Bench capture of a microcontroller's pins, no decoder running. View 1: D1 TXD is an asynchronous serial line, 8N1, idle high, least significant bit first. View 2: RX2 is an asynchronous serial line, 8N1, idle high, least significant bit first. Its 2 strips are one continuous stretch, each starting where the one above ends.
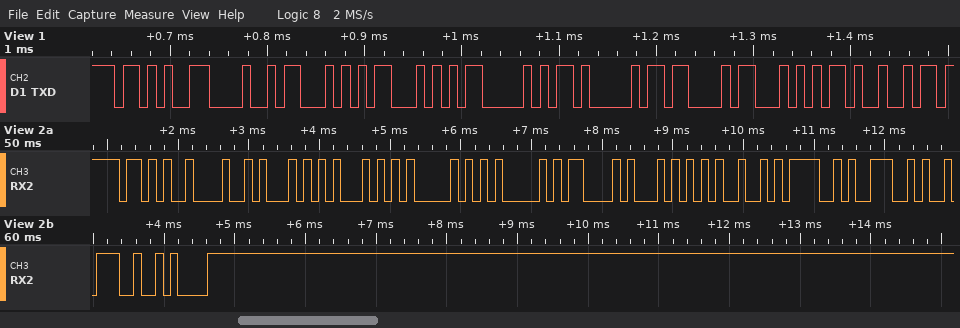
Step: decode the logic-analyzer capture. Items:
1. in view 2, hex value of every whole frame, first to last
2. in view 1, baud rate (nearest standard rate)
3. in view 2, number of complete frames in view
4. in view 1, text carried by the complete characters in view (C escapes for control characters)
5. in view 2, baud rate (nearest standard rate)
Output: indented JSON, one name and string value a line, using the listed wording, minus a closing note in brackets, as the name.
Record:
{
  "in view 2, hex value of every whole frame, first to last": "0x2B 0x48 0x54 0x54 0x50 0x41 0x43 0x54 0x49 0x4F 0x4E 0x3A 0x0A",
  "in view 1, baud rate": "115200 baud",
  "in view 2, number of complete frames in view": "13",
  "in view 1, text carried by the complete characters in view": "\"+HTTPACTI\"",
  "in view 2, baud rate": "9600 baud"
}
